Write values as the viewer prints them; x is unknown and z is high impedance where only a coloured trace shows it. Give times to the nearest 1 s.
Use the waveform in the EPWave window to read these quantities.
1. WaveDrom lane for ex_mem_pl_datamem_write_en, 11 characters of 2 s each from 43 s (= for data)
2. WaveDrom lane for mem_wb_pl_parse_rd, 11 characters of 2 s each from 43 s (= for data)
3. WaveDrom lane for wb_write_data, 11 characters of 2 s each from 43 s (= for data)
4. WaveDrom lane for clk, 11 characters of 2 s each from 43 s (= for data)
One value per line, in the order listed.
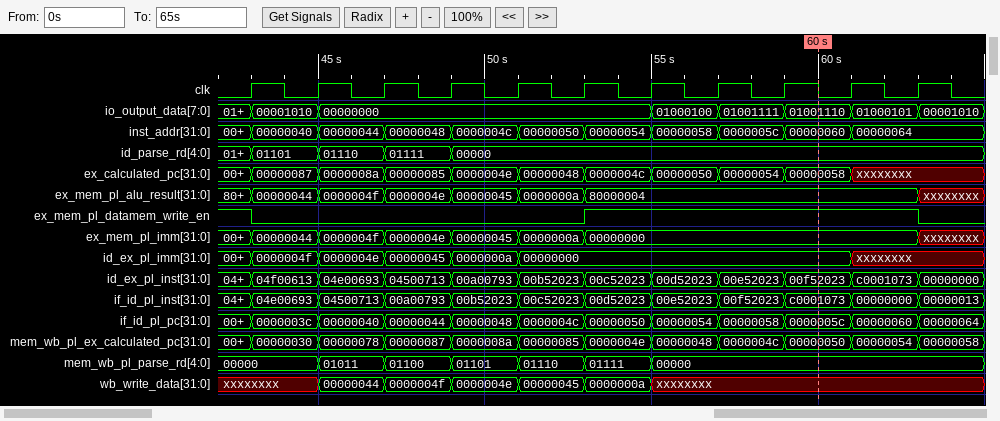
{name: 'ex_mem_pl_datamem_write_en', wave: '0....1....0'}
{name: 'mem_wb_pl_parse_rd', wave: '=======....', data: '00000 01011 01100 01101 01110 01111 00000'}
{name: 'wb_write_data', wave: 'x=====x....', data: '00000044 0000004f 0000004e 00000045 0000000a'}
{name: 'clk', wave: 'p..........'}
